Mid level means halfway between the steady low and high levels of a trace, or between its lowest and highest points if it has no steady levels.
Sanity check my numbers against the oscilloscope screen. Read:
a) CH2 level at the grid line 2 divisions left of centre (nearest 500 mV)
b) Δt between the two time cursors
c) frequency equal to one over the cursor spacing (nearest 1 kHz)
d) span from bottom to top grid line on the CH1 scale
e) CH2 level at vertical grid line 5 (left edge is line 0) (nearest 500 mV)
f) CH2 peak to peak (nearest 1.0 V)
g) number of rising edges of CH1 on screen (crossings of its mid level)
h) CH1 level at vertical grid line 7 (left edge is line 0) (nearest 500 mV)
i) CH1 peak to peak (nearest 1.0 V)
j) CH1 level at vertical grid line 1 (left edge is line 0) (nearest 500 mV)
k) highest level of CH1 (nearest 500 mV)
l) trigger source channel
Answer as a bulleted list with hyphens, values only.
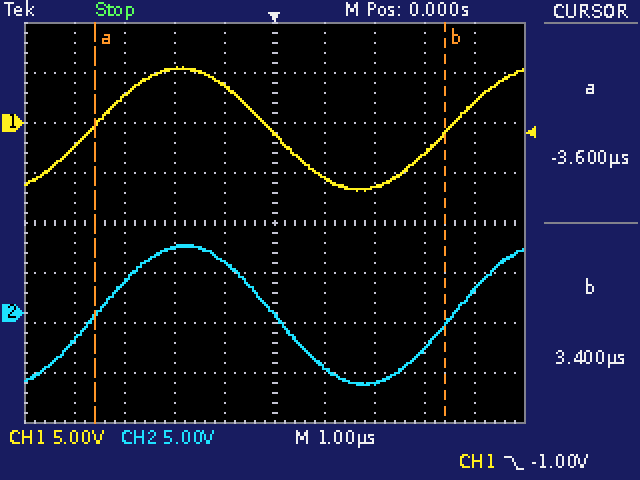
- 6.5 V
- 7.0 µs
- 143 kHz
- 40 V
- 0.0 V
- 14.0 V
- 2
- -6.5 V
- 12.0 V
- -2.5 V
- 5.5 V
- CH1
